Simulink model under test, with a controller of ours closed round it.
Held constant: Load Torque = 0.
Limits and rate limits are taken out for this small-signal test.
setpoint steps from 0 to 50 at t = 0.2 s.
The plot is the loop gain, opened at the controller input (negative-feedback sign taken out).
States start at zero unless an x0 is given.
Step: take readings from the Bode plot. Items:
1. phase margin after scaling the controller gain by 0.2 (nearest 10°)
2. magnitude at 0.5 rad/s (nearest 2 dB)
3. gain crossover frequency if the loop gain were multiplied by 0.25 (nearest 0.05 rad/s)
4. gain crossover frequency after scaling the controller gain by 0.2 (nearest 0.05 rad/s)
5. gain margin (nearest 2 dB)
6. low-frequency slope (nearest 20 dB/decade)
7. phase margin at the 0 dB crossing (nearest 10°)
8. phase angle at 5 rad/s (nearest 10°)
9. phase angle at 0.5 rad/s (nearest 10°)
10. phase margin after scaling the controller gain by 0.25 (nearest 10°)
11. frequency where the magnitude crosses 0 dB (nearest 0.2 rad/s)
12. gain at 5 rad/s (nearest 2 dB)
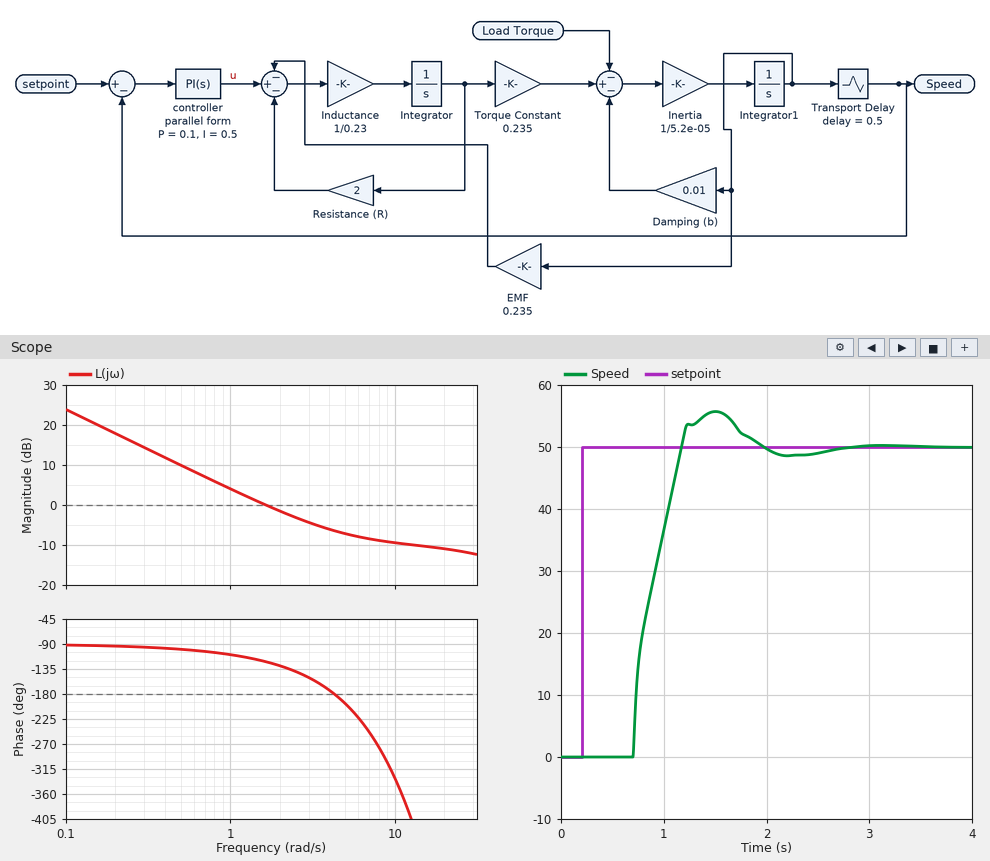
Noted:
80°
10 dB
0.40 rad/s
0.30 rad/s
6 dB
-20 dB/decade
60°
-200°
-100°
80°
1.6 rad/s
-8 dB
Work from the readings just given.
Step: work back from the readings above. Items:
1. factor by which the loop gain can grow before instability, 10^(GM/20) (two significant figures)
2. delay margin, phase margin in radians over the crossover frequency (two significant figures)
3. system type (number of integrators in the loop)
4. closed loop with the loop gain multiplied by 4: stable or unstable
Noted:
2.0
0.65 s
1
unstable
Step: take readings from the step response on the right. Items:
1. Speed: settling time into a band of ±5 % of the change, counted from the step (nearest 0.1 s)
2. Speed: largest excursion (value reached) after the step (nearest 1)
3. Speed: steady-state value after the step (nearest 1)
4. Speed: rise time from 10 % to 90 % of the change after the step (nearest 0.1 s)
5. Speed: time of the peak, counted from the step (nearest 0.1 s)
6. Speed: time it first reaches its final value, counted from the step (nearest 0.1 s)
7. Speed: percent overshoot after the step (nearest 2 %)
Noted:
1.5 s
56
50
0.4 s
1.3 s
1.0 s
12 %
